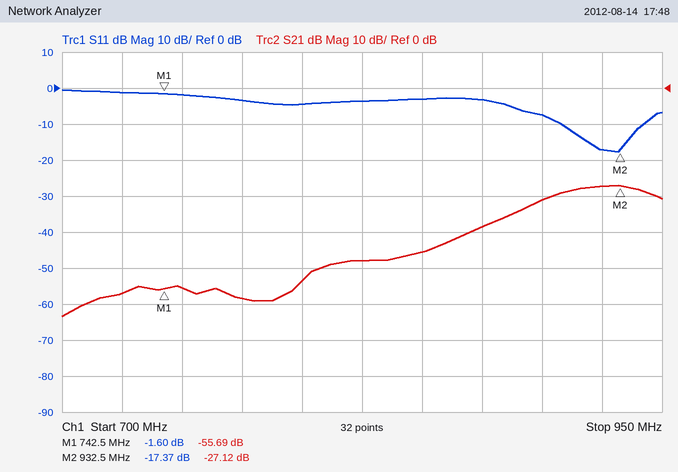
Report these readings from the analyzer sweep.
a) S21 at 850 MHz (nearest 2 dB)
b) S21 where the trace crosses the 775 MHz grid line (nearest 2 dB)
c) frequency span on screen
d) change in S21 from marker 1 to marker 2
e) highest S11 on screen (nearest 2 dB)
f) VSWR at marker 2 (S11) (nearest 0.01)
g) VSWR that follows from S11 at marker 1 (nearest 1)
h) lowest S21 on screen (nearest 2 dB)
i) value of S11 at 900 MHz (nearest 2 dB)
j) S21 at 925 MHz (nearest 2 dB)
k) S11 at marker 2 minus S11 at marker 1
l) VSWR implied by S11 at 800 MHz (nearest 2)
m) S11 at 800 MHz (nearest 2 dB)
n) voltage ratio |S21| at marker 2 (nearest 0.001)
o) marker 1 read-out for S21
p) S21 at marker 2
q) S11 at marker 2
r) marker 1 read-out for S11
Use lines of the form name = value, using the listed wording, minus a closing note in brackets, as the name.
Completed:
S21 at 850 MHz = -46 dB
S21 where the trace crosses the 775 MHz grid line = -58 dB
frequency span on screen = 250 MHz
change in S21 from marker 1 to marker 2 = 28.57 dB
highest S11 on screen = 0 dB
VSWR at marker 2 (S11) = 1.31
VSWR that follows from S11 at marker 1 = 11
lowest S21 on screen = -64 dB
value of S11 at 900 MHz = -8 dB
S21 at 925 MHz = -28 dB
S11 at marker 2 minus S11 at marker 1 = -15.77 dB
VSWR implied by S11 at 800 MHz = 4
S11 at 800 MHz = -4 dB
voltage ratio |S21| at marker 2 = 0.044
marker 1 read-out for S21 = -55.69 dB
S21 at marker 2 = -27.12 dB
S11 at marker 2 = -17.37 dB
marker 1 read-out for S11 = -1.60 dB
